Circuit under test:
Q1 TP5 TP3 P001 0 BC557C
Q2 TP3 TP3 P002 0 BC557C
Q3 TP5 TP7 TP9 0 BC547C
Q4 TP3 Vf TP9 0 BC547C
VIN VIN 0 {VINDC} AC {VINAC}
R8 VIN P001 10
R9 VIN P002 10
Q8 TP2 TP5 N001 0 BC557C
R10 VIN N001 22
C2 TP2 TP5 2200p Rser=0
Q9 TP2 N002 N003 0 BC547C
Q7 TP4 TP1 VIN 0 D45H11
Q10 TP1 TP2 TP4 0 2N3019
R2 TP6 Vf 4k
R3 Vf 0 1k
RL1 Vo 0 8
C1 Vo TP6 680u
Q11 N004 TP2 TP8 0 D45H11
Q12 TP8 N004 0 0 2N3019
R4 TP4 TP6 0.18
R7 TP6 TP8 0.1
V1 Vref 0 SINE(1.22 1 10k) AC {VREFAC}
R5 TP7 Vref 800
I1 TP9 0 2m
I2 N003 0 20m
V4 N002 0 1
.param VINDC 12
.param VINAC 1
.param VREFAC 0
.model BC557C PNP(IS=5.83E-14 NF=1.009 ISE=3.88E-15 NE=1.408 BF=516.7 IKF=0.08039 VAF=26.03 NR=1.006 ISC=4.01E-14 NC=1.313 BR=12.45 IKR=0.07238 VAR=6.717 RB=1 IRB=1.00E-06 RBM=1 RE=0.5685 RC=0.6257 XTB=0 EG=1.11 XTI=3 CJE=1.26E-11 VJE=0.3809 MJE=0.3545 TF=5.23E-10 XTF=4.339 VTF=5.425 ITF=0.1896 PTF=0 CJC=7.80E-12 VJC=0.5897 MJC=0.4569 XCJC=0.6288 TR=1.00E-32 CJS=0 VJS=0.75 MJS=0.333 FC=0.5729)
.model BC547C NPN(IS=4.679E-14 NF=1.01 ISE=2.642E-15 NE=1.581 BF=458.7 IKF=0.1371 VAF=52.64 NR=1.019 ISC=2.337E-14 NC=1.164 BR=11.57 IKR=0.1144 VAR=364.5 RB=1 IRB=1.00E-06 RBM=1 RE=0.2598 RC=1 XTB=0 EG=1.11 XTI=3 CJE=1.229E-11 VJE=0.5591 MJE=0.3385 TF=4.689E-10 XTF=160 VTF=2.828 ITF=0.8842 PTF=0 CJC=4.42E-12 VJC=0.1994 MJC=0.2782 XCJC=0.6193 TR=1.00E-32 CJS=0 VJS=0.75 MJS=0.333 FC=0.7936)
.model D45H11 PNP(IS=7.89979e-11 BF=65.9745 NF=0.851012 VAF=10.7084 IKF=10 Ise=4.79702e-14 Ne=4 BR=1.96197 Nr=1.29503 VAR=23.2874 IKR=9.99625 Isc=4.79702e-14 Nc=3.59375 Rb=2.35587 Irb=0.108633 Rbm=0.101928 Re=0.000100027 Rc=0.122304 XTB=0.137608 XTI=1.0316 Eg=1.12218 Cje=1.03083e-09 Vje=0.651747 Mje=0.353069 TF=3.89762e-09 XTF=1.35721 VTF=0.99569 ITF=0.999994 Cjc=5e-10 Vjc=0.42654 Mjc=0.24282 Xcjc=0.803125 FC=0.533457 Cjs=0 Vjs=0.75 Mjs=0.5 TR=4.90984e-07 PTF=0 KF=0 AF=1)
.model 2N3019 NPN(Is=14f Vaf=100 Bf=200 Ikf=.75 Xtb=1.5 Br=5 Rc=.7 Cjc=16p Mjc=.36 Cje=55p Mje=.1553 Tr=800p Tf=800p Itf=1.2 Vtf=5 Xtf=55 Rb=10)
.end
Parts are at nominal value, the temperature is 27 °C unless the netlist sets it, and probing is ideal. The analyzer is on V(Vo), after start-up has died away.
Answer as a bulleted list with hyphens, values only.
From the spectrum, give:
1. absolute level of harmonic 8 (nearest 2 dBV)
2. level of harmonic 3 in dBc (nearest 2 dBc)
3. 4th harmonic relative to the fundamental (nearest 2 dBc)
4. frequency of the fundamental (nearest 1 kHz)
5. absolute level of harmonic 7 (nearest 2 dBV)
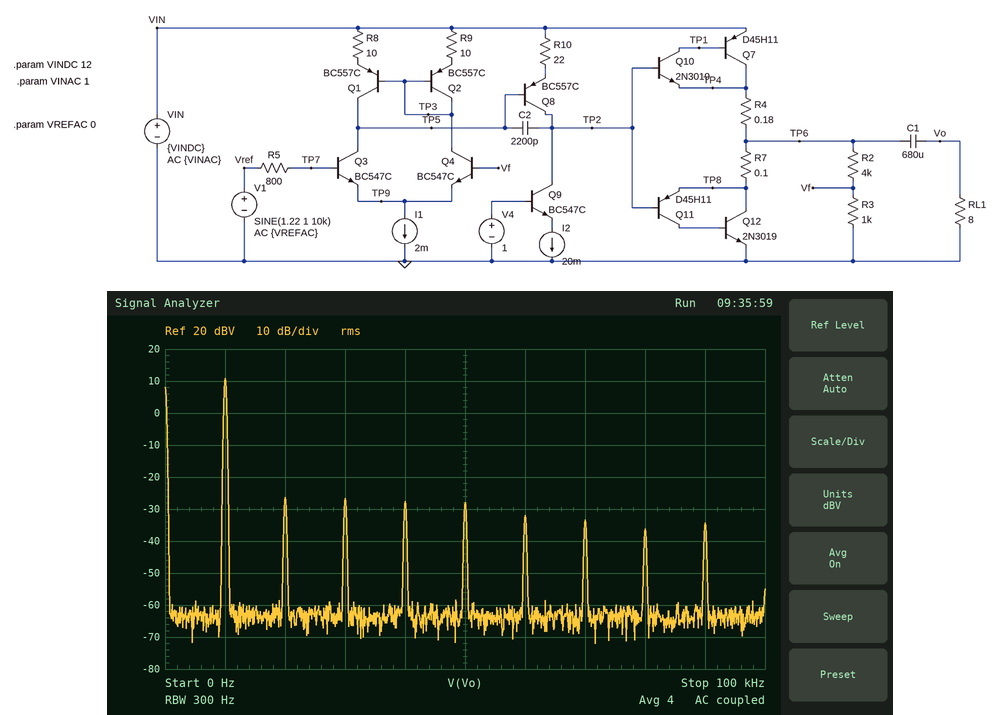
- -36 dBV
- -38 dBc
- -38 dBc
- 10 kHz
- -34 dBV
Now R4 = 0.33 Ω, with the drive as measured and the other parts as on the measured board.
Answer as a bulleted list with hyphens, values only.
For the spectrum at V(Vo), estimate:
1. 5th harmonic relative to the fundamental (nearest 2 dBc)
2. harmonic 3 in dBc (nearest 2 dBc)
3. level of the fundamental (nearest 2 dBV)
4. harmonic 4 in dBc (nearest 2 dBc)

- -38 dBc
- -36 dBc
- 10 dBV
- -36 dBc
